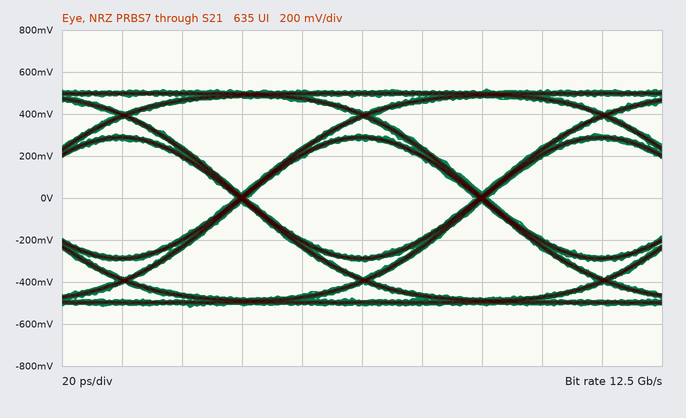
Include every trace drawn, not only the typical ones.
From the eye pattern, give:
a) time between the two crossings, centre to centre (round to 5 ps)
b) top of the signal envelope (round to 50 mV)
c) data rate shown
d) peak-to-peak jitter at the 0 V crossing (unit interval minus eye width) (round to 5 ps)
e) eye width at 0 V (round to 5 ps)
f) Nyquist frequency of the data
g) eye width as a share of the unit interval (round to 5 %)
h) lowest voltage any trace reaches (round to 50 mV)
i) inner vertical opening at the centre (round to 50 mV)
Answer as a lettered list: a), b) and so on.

a) 80 ps
b) 500 mV
c) 12.5 Gb/s
d) 5 ps
e) 75 ps
f) 6.25 GHz
g) 95 %
h) -500 mV
i) 550 mV
